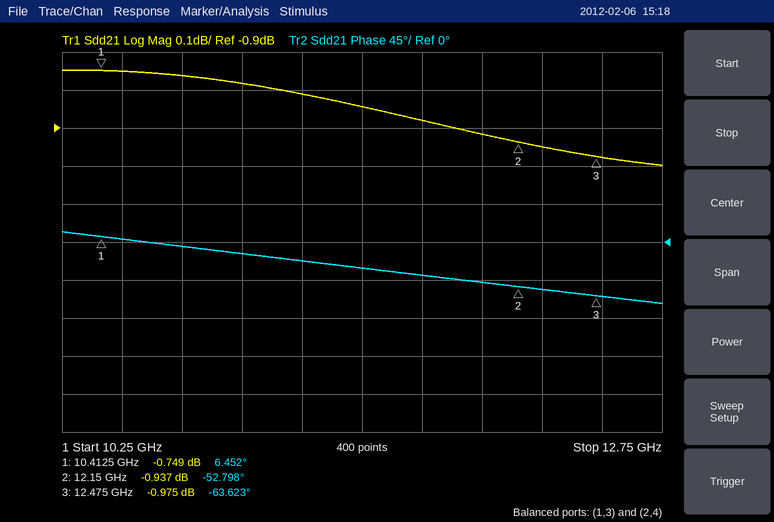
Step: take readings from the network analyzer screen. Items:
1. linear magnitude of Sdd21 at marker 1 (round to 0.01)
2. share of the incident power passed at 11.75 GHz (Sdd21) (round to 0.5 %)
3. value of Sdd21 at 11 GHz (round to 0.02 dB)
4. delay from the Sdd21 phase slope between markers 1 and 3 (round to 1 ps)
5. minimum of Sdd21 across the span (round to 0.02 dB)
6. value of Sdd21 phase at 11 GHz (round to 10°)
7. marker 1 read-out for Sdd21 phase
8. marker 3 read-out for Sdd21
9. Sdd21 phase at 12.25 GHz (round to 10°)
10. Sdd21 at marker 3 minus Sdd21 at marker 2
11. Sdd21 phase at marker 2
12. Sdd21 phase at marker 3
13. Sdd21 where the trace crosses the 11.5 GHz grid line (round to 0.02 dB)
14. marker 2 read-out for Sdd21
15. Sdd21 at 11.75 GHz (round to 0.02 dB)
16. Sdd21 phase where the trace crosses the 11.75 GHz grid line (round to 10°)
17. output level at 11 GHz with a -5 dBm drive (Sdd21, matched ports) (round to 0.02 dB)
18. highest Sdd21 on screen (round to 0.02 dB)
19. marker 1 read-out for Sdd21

0.92
81.5 %
-0.78 dB
94 ps
-1.00 dB
-10°
6.452°
-0.975 dB
-60°
-0.038 dB
-52.798°
-63.623°
-0.84 dB
-0.937 dB
-0.88 dB
-40°
-5.78 dBm
-0.74 dB
-0.749 dB
